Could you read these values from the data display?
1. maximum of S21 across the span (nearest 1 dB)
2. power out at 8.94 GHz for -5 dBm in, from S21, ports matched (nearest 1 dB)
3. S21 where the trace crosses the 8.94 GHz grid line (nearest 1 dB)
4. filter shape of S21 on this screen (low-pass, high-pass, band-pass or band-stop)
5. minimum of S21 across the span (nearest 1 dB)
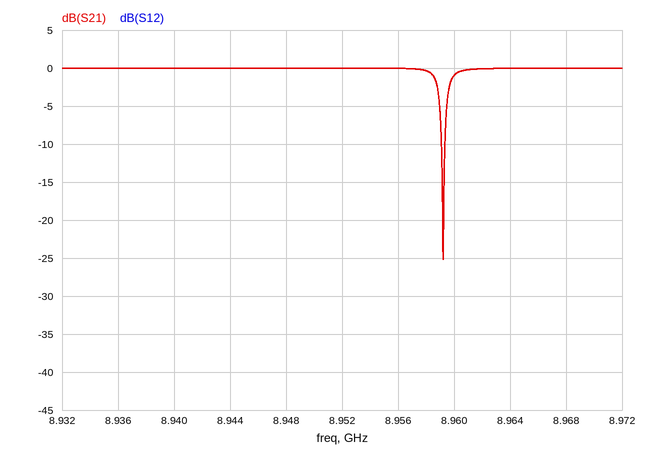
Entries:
0 dB
-5 dBm
0 dB
band-stop
-25 dB
